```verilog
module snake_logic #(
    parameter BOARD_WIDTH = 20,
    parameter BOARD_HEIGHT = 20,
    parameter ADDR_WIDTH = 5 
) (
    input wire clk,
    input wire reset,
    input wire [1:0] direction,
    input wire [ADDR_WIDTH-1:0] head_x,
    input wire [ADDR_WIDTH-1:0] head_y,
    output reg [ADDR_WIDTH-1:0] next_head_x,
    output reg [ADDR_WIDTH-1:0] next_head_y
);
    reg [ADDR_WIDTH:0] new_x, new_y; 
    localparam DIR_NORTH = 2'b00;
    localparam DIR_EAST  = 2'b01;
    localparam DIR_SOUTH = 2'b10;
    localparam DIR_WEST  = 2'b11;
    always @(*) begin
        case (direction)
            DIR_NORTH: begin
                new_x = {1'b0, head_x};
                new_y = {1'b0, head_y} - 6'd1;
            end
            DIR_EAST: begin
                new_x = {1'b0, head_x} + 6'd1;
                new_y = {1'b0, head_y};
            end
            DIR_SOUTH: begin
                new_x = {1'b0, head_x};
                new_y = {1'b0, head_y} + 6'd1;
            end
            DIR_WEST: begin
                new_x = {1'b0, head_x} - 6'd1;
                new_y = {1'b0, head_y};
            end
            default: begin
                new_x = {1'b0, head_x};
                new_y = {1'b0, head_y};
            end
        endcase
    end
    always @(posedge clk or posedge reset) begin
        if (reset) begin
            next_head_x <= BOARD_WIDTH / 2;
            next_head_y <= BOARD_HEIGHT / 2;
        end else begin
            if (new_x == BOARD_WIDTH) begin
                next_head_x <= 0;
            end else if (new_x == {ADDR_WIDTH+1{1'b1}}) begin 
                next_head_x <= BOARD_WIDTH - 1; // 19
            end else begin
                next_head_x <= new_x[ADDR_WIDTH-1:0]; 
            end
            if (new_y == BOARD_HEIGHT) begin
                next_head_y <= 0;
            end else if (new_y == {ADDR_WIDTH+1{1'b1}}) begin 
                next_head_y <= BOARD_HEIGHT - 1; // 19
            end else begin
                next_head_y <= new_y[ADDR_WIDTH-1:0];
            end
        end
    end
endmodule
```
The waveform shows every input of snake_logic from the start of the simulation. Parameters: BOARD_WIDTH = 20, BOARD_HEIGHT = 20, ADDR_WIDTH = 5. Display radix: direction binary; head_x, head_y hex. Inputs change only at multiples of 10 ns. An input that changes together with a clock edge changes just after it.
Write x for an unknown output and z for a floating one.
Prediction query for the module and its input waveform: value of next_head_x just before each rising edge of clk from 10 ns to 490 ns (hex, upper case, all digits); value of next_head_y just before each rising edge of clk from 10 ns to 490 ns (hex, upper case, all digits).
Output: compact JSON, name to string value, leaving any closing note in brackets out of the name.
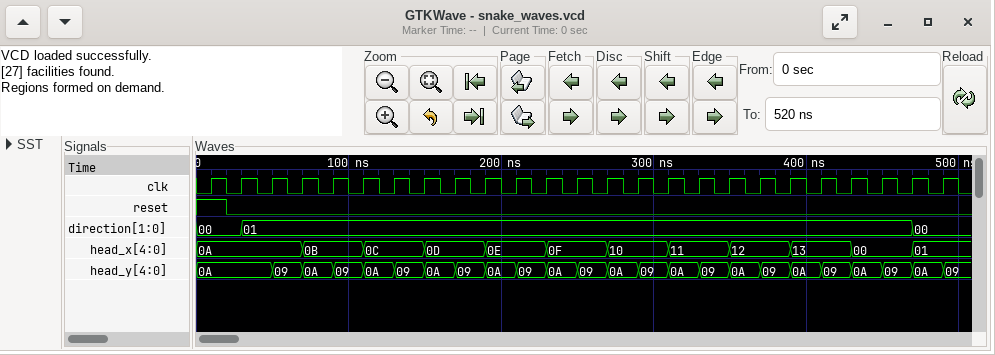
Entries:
{"value of next_head_x just before each rising edge of clk from 10 ns to 490 ns": "0A, 0A, 0A, 0B, 0B, 0C, 0C, 0D, 0D, 0E, 0E, 0F, 0F, 10, 10, 11, 11, 12, 12, 13, 13, 00, 00, 01, 01", "value of next_head_y just before each rising edge of clk from 10 ns to 490 ns": "0A, 0A, 09, 0A, 09, 0A, 09, 0A, 09, 0A, 09, 0A, 09, 0A, 09, 0A, 09, 0A, 09, 0A, 09, 0A, 09, 0A, 09"}
